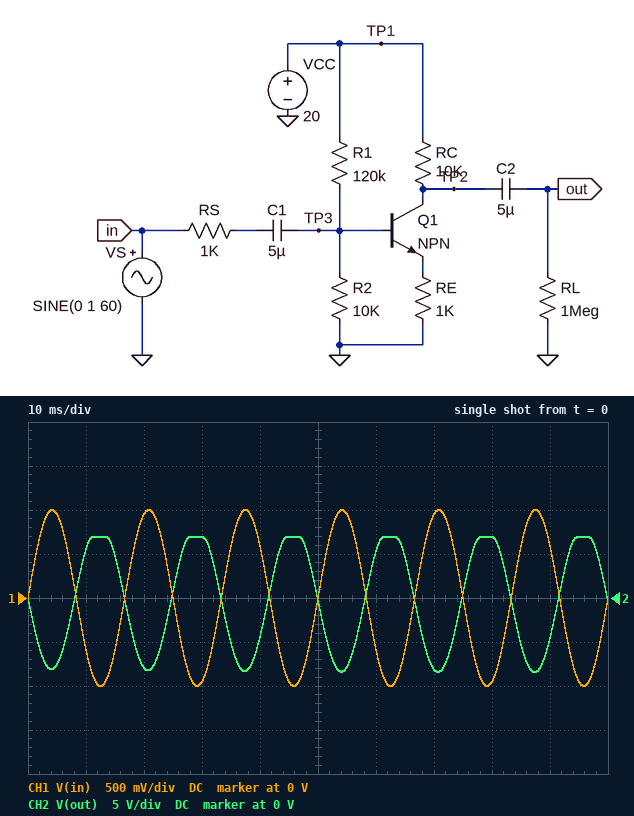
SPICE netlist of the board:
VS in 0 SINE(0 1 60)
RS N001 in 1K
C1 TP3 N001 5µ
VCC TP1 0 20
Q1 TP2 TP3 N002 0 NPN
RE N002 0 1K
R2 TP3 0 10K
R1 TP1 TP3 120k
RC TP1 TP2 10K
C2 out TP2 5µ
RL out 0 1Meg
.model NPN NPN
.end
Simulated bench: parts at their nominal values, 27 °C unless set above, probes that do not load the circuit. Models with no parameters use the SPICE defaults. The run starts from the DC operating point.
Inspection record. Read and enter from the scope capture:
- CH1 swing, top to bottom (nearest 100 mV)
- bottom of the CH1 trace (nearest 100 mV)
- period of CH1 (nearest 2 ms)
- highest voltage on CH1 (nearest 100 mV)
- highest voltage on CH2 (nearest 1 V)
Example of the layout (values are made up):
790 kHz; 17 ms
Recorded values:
2.0 V; -1.0 V; 16 ms; 1.0 V; 7 V
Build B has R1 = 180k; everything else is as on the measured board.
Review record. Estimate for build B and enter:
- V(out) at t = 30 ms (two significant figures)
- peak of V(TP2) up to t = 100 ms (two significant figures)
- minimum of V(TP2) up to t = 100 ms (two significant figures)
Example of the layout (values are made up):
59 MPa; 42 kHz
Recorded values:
2.8 V; 20 V; 8.9 V
